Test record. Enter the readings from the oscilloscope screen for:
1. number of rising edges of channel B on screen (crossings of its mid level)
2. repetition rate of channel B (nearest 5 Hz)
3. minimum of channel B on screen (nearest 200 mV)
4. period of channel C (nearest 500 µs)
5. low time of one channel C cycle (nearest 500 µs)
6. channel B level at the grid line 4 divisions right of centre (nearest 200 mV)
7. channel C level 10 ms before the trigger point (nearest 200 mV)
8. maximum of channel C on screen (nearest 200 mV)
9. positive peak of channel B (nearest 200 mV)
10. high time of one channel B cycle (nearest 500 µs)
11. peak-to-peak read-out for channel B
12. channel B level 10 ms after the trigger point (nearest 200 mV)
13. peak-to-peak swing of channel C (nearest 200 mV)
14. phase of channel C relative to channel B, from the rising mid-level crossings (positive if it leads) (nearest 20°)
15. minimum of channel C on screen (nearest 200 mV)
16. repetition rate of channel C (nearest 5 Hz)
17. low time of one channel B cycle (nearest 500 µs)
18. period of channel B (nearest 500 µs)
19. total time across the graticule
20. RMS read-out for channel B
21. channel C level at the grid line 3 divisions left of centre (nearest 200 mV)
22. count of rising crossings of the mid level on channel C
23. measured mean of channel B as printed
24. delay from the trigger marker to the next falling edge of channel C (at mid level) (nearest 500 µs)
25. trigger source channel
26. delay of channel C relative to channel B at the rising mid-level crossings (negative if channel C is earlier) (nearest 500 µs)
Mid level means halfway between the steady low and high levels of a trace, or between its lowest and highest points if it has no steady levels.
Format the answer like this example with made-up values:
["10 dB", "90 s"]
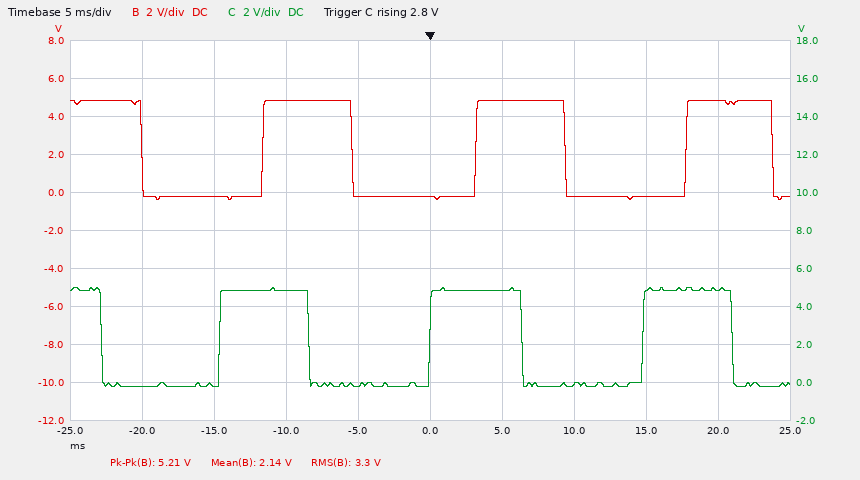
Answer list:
["3", "70 Hz", "-400 mV", "14.5 ms", "8.5 ms", "4.8 V", "4.8 V", "5.0 V", "4.8 V", "6.0 ms", "5.21 V", "-200 mV", "5.2 V", "+80°", "-200 mV", "70 Hz", "8.5 ms", "14.5 ms", "50 ms", "3.3 V", "-200 mV", "3", "2.14 V", "6.5 ms", "channel C", "-3.0 ms"]
